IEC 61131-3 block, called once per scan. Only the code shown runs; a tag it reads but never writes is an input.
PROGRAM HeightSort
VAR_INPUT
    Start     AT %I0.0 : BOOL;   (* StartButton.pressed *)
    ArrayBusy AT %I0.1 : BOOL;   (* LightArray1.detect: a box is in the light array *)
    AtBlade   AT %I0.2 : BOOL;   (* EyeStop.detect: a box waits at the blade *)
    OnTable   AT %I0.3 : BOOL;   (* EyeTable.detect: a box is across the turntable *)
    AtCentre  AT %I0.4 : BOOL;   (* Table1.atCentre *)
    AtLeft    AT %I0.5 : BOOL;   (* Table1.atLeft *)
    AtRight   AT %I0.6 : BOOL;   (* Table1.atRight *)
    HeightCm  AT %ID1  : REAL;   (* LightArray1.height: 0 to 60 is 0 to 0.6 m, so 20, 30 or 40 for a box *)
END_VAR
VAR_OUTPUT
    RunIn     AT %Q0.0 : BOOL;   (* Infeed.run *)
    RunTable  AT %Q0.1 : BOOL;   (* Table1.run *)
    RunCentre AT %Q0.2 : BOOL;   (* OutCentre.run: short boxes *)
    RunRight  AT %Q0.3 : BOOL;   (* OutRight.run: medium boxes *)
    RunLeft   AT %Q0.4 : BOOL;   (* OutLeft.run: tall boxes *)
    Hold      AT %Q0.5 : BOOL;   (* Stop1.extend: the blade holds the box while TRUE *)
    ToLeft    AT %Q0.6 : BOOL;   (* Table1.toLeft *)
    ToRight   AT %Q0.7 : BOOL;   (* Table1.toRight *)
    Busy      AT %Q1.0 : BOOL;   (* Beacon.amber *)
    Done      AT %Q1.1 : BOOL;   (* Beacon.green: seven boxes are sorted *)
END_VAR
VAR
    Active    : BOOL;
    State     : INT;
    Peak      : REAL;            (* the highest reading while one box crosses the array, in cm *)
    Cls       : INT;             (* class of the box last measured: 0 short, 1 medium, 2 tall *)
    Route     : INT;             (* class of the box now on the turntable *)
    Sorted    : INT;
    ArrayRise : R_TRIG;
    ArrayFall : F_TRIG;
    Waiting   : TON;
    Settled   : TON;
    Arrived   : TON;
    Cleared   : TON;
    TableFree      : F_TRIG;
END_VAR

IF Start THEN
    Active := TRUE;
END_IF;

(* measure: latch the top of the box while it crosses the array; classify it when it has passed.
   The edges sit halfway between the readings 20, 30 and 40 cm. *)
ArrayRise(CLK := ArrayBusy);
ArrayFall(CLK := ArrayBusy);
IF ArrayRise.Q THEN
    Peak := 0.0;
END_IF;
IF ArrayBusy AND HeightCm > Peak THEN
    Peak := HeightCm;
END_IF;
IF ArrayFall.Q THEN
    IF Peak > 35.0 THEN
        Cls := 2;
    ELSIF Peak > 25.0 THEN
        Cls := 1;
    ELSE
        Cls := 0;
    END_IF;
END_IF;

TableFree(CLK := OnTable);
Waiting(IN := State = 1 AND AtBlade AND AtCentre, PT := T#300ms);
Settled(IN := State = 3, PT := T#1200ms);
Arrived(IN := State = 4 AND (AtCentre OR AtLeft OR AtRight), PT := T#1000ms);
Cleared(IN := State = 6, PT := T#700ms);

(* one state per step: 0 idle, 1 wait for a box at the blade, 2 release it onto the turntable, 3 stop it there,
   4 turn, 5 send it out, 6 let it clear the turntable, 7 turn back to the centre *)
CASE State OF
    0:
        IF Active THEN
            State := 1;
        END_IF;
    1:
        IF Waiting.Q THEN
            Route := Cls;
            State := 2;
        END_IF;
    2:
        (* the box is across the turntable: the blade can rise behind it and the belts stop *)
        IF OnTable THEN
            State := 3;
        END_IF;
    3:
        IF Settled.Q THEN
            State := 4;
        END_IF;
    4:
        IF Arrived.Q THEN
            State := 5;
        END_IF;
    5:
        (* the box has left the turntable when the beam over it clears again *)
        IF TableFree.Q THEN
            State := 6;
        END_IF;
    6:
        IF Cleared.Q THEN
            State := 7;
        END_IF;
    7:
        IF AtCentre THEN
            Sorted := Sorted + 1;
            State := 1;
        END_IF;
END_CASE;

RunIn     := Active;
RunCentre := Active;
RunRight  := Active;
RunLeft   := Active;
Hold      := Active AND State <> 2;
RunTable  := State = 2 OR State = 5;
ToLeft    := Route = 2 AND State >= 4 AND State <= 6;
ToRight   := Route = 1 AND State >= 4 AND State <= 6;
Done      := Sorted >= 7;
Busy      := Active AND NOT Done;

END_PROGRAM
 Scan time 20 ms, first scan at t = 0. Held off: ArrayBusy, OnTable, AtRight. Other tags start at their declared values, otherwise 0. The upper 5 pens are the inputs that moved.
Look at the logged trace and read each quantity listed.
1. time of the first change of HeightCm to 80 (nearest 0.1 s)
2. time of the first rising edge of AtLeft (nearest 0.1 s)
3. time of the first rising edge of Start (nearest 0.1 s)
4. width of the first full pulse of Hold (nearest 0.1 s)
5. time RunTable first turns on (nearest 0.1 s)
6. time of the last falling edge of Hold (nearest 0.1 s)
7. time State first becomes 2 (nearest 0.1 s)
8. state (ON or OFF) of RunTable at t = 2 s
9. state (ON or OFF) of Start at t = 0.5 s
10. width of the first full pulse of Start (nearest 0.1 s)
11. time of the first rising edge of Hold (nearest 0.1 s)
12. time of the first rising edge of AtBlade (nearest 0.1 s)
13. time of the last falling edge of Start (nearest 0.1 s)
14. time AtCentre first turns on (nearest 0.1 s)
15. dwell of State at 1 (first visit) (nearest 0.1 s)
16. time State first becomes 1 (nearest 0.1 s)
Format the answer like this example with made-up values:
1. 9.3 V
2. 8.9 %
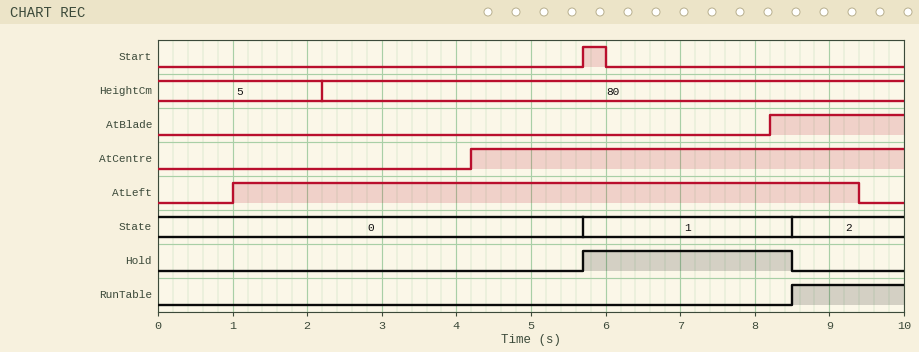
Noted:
1. 2.2 s
2. 1.0 s
3. 5.7 s
4. 2.8 s
5. 8.5 s
6. 8.5 s
7. 8.5 s
8. OFF
9. OFF
10. 0.3 s
11. 5.7 s
12. 8.2 s
13. 6.0 s
14. 4.2 s
15. 2.8 s
16. 5.7 s
